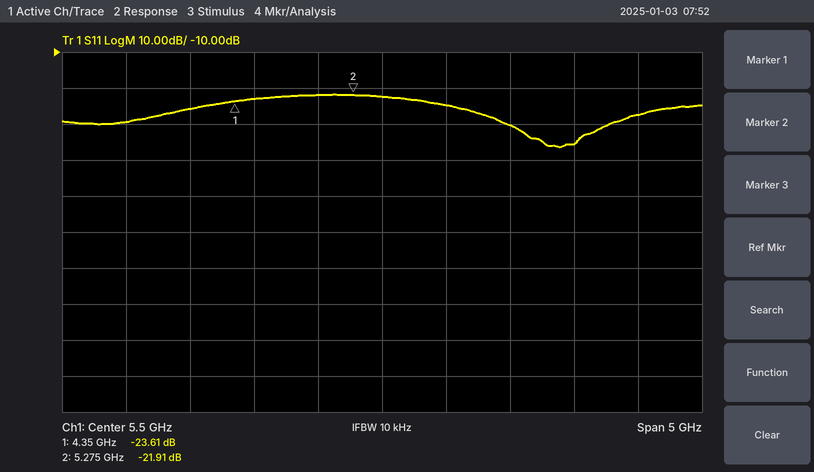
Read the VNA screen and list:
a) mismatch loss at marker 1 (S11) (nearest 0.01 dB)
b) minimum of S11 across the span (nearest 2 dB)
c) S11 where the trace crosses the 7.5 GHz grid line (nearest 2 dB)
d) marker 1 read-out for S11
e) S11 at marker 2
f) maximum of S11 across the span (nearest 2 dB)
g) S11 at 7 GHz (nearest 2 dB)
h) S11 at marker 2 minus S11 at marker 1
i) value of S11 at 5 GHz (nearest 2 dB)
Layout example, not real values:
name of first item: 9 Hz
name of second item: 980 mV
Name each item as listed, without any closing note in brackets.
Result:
mismatch loss at marker 1 (S11): 0.02 dB
minimum of S11 across the span: -36 dB
S11 where the trace crosses the 7.5 GHz grid line: -28 dB
marker 1 read-out for S11: -23.61 dB
S11 at marker 2: -21.91 dB
maximum of S11 across the span: -22 dB
S11 at 7 GHz: -36 dB
S11 at marker 2 minus S11 at marker 1: 1.70 dB
value of S11 at 5 GHz: -22 dB
